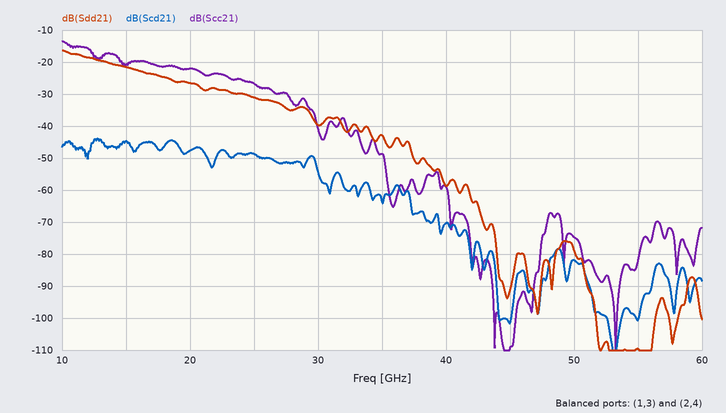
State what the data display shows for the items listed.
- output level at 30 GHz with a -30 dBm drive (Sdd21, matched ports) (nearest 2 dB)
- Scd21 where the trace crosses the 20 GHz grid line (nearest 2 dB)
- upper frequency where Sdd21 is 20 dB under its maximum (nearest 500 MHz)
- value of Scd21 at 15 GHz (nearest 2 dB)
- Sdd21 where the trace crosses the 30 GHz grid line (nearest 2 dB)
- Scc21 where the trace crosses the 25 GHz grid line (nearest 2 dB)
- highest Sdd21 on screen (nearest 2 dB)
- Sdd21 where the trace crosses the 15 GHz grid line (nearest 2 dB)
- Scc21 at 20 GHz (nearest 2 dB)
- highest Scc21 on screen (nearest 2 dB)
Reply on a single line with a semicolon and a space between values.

-70 dBm; -48 dB; 29.5 GHz; -44 dB; -40 dB; -26 dB; -16 dB; -22 dB; -22 dB; -14 dB
